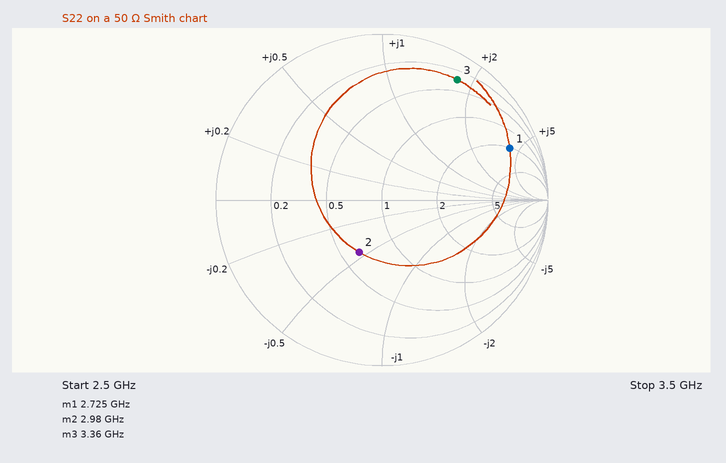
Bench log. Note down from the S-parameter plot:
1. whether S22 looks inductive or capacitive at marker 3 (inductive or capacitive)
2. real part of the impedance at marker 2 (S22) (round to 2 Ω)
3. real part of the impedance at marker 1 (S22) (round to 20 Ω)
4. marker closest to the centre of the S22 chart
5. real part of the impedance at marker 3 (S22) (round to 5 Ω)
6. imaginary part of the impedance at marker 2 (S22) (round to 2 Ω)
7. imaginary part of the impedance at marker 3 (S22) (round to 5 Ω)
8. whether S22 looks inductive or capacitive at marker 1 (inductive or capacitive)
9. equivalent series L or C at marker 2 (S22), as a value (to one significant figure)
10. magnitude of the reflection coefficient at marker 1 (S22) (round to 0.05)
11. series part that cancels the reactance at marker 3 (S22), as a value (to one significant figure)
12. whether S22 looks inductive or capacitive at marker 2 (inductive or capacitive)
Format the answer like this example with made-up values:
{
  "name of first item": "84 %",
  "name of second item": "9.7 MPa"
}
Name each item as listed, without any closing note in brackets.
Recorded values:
{
  "whether S22 looks inductive or capacitive at marker 3": "inductive",
  "real part of the impedance at marker 2 (S22)": "32 Ω",
  "real part of the impedance at marker 1 (S22)": "100 Ω",
  "marker closest to the centre of the S22 chart": "marker 2",
  "real part of the impedance at marker 3 (S22)": "15 Ω",
  "imaginary part of the impedance at marker 2 (S22)": "-22 Ω",
  "imaginary part of the impedance at marker 3 (S22)": "+90 Ω",
  "whether S22 looks inductive or capacitive at marker 1": "inductive",
  "equivalent series L or C at marker 2 (S22), as a value": "2 pF",
  "magnitude of the reflection coefficient at marker 1 (S22)": "0.85",
  "series part that cancels the reactance at marker 3 (S22), as a value": "500 fF",
  "whether S22 looks inductive or capacitive at marker 2": "capacitive"
}
